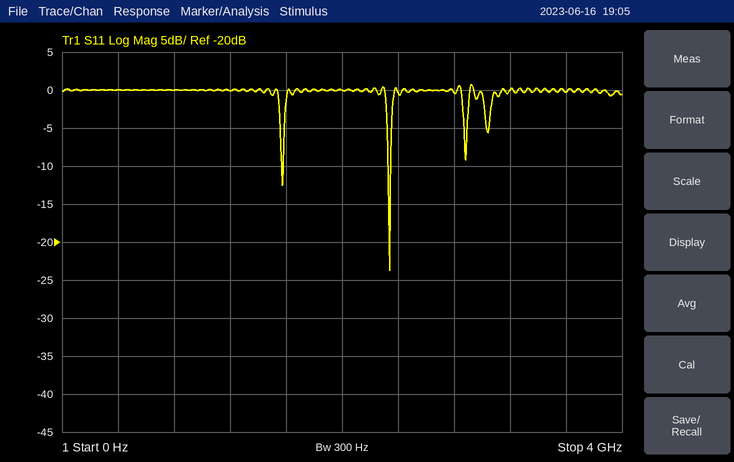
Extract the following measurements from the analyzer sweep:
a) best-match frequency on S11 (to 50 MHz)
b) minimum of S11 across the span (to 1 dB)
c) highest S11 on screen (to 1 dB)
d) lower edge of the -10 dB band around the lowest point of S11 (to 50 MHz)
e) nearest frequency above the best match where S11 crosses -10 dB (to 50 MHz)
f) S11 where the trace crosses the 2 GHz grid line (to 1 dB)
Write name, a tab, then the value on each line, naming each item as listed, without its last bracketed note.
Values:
best-match frequency on S11	2.35 GHz
minimum of S11 across the span	-24 dB
highest S11 on screen	1 dB
lower edge of the -10 dB band around the lowest point of S11	2.35 GHz
nearest frequency above the best match where S11 crosses -10 dB	2.35 GHz
S11 where the trace crosses the 2 GHz grid line	0 dB
